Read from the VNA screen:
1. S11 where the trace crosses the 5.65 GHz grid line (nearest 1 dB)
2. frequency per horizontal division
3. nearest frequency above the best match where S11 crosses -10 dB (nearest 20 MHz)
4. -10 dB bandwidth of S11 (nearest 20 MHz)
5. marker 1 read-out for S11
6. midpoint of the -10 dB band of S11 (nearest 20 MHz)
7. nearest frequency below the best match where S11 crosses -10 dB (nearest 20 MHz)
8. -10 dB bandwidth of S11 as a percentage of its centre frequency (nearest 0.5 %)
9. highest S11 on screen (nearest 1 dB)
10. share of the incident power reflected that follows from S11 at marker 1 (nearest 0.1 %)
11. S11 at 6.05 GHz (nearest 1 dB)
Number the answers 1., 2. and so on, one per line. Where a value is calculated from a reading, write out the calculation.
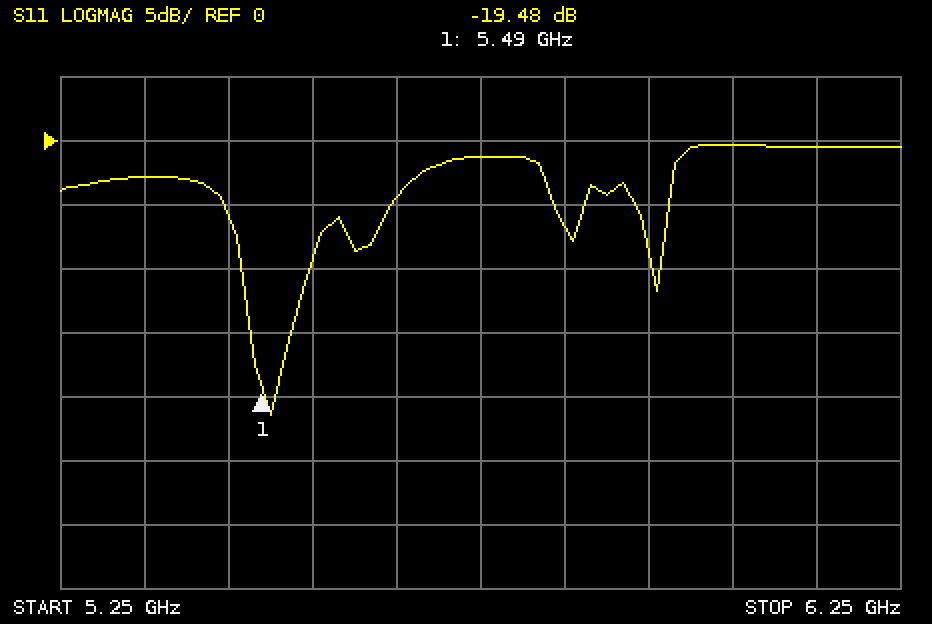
1. -4 dB
2. 100 MHz
3. 5.54 GHz
4. 5.54 GHz − 5.46 GHz = 80 MHz
5. -19.48 dB
6. 5.50 GHz
7. 5.46 GHz
8. 80 MHz / 5.5 GHz ≈ 1.5 %
9. 0 dB
10. 10^(-19.48/10) ≈ 1.1 %
11. 0 dB
